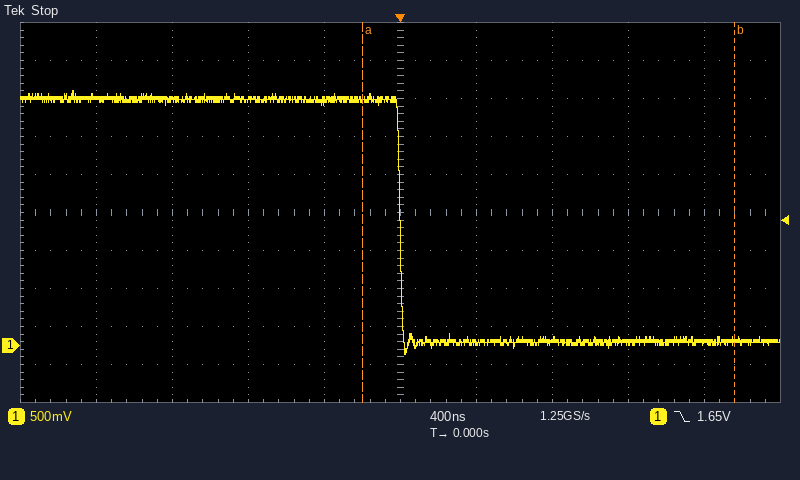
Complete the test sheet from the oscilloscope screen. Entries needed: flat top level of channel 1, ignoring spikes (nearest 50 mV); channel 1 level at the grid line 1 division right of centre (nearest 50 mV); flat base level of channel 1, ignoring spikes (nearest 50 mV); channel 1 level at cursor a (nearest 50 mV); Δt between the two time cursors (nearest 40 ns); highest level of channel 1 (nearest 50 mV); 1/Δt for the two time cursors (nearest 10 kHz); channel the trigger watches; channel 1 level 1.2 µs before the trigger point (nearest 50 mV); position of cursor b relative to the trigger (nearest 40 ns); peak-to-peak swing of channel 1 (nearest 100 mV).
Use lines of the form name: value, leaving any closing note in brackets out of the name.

flat top level of channel 1, ignoring spikes: 3.25 V
channel 1 level at the grid line 1 division right of centre: 50 mV
flat base level of channel 1, ignoring spikes: 50 mV
channel 1 level at cursor a: 3.25 V
Δt between the two time cursors: 1.96 µs
highest level of channel 1: 3.35 V
1/Δt for the two time cursors: 510 kHz
channel the trigger watches: channel 1
channel 1 level 1.2 µs before the trigger point: 3.25 V
position of cursor b relative to the trigger: +1.76 µs
peak-to-peak swing of channel 1: 3.50 V
